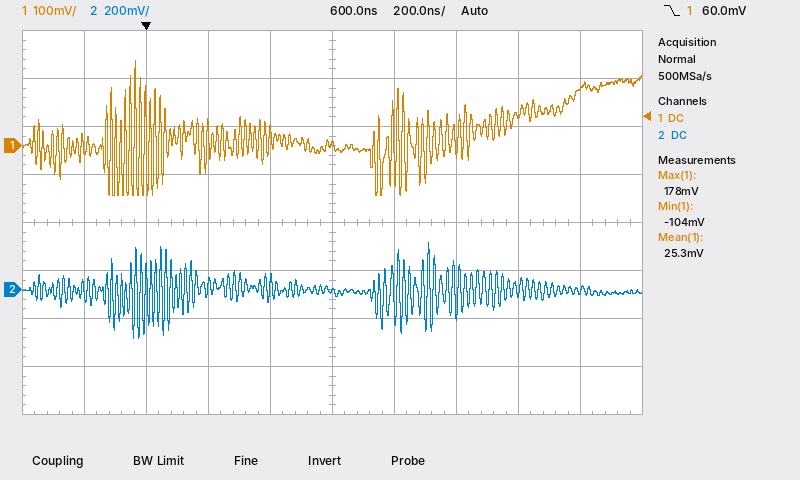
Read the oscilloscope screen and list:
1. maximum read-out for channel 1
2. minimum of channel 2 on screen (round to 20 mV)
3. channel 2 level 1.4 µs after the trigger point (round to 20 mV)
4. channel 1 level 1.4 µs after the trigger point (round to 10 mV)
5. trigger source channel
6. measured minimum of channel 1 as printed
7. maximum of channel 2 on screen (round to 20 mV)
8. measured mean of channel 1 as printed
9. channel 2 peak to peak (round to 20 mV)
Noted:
178 mV
-200 mV
0 mV
120 mV
channel 1
-104 mV
200 mV
25.3 mV
400 mV
